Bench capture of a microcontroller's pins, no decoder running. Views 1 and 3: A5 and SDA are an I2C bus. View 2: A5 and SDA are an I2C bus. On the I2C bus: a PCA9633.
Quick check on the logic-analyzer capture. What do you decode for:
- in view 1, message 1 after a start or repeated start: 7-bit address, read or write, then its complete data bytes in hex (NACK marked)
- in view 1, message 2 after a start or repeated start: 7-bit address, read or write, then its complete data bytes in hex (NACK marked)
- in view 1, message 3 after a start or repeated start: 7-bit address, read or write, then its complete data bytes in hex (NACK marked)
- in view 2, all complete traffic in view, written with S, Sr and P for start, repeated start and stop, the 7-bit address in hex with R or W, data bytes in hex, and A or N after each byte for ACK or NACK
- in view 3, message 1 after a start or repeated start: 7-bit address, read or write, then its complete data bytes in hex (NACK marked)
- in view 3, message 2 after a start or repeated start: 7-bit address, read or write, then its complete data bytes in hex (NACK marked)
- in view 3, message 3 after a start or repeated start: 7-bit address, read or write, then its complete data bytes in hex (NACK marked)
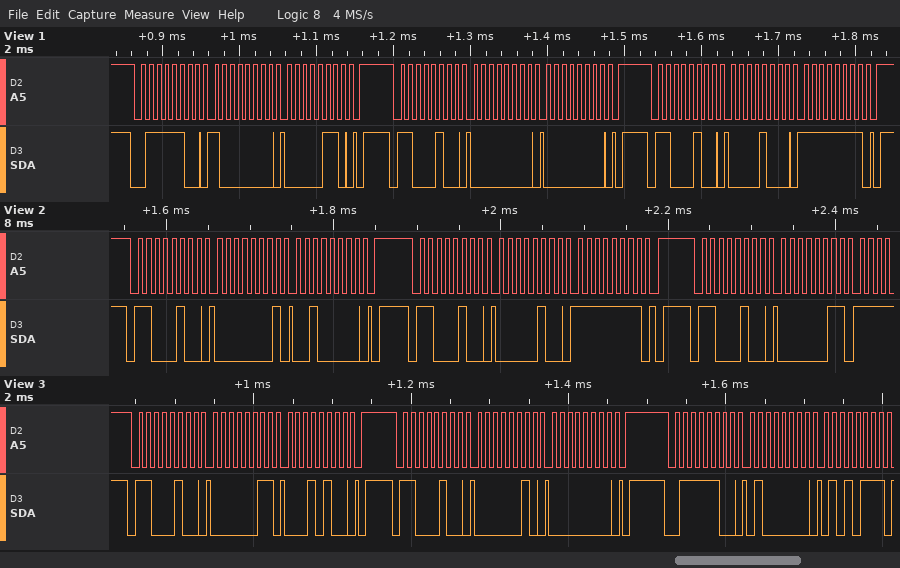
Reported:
0x3E write: 80 06
0x62 write: 00 00
0x62 write: 08 FF
S 62W A 01 A 20 A P S 62W A 04 A FF A P S 62W A 03 A
0x62 write: 03 14
0x62 write: 02 00
0x3E write: 40 57
